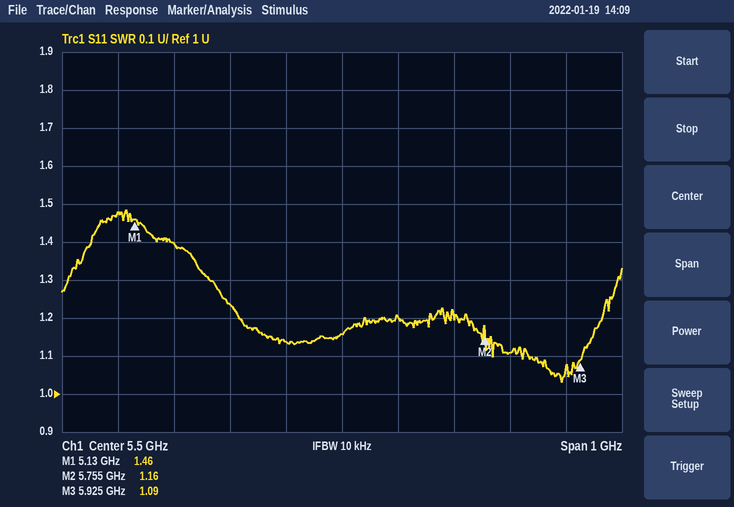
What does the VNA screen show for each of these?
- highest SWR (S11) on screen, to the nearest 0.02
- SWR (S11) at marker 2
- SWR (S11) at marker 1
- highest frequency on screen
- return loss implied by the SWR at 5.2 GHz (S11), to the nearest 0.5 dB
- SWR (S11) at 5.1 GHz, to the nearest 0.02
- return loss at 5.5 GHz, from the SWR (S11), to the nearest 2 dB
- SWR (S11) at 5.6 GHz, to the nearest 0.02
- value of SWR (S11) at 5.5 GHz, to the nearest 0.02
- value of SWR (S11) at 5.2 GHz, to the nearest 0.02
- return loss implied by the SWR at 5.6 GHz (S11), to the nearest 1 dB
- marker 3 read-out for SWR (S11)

1.48
1.16
1.46
6 GHz
15.5 dB
1.48
22 dB
1.20
1.16
1.40
21 dB
1.09
